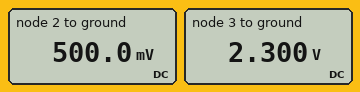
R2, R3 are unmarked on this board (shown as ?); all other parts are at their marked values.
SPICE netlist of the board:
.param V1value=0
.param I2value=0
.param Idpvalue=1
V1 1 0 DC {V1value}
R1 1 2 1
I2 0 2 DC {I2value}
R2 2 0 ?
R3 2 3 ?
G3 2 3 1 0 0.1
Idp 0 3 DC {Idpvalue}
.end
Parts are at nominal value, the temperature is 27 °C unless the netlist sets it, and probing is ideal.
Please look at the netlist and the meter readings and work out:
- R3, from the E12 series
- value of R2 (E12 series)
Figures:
1.8 Ω
1 Ω
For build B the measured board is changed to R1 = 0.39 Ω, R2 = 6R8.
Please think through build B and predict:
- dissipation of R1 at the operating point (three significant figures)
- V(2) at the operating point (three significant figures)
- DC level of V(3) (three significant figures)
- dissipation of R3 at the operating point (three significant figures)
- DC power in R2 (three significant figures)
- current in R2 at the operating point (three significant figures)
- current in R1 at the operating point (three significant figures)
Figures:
349 mW
369 mV
2.17 V
1.80 W
20.0 mW
54.2 mA
946 mA
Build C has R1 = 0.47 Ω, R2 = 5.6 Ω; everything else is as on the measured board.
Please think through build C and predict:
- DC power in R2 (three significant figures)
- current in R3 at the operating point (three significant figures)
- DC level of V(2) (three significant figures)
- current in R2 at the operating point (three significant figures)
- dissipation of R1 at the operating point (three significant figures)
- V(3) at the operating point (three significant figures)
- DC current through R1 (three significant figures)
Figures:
33.6 mW
1.00 A
434 mV
77.4 mA
400 mW
2.23 V
923 mA
